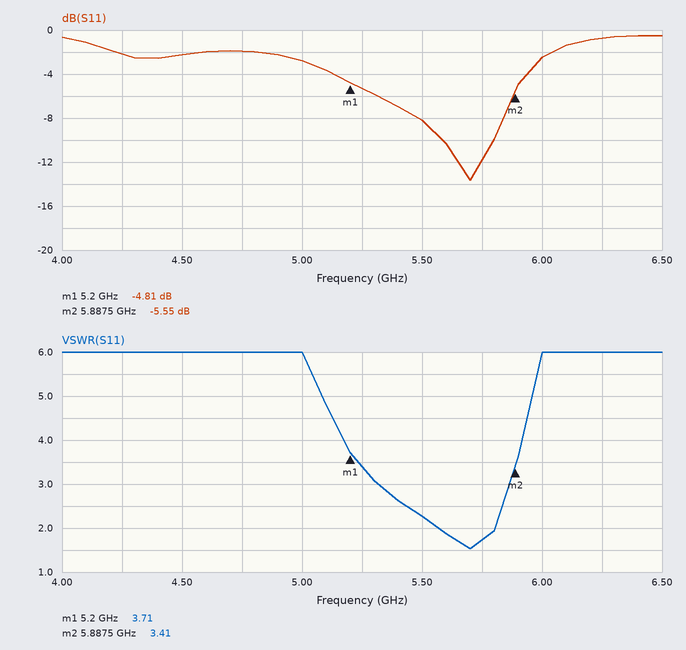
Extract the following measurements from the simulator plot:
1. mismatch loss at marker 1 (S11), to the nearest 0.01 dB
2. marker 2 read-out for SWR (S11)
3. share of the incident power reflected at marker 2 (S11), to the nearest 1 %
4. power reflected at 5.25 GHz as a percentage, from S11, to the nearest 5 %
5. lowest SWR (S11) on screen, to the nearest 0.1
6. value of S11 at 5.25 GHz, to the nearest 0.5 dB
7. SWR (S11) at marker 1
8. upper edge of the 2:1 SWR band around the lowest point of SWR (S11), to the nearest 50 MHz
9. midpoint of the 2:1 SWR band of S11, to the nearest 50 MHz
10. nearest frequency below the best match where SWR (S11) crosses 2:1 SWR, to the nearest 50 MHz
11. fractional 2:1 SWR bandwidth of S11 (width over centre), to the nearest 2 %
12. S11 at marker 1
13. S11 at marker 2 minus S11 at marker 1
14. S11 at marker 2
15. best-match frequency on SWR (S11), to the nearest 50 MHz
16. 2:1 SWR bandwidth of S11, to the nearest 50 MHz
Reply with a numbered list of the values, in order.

1. 1.74 dB
2. 3.41
3. 28 %
4. 30 %
5. 1.5
6. -5.5 dB
7. 3.71
8. 5.80 GHz
9. 5.70 GHz
10. 5.55 GHz
11. 4 %
12. -4.81 dB
13. -0.74 dB
14. -5.55 dB
15. 5.70 GHz
16. 250 MHz
